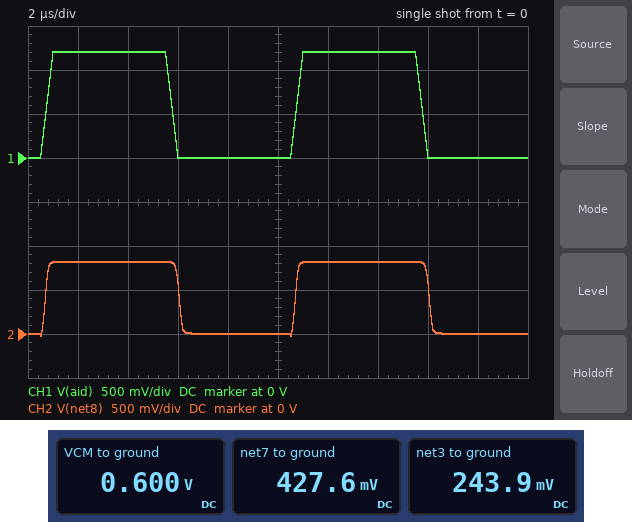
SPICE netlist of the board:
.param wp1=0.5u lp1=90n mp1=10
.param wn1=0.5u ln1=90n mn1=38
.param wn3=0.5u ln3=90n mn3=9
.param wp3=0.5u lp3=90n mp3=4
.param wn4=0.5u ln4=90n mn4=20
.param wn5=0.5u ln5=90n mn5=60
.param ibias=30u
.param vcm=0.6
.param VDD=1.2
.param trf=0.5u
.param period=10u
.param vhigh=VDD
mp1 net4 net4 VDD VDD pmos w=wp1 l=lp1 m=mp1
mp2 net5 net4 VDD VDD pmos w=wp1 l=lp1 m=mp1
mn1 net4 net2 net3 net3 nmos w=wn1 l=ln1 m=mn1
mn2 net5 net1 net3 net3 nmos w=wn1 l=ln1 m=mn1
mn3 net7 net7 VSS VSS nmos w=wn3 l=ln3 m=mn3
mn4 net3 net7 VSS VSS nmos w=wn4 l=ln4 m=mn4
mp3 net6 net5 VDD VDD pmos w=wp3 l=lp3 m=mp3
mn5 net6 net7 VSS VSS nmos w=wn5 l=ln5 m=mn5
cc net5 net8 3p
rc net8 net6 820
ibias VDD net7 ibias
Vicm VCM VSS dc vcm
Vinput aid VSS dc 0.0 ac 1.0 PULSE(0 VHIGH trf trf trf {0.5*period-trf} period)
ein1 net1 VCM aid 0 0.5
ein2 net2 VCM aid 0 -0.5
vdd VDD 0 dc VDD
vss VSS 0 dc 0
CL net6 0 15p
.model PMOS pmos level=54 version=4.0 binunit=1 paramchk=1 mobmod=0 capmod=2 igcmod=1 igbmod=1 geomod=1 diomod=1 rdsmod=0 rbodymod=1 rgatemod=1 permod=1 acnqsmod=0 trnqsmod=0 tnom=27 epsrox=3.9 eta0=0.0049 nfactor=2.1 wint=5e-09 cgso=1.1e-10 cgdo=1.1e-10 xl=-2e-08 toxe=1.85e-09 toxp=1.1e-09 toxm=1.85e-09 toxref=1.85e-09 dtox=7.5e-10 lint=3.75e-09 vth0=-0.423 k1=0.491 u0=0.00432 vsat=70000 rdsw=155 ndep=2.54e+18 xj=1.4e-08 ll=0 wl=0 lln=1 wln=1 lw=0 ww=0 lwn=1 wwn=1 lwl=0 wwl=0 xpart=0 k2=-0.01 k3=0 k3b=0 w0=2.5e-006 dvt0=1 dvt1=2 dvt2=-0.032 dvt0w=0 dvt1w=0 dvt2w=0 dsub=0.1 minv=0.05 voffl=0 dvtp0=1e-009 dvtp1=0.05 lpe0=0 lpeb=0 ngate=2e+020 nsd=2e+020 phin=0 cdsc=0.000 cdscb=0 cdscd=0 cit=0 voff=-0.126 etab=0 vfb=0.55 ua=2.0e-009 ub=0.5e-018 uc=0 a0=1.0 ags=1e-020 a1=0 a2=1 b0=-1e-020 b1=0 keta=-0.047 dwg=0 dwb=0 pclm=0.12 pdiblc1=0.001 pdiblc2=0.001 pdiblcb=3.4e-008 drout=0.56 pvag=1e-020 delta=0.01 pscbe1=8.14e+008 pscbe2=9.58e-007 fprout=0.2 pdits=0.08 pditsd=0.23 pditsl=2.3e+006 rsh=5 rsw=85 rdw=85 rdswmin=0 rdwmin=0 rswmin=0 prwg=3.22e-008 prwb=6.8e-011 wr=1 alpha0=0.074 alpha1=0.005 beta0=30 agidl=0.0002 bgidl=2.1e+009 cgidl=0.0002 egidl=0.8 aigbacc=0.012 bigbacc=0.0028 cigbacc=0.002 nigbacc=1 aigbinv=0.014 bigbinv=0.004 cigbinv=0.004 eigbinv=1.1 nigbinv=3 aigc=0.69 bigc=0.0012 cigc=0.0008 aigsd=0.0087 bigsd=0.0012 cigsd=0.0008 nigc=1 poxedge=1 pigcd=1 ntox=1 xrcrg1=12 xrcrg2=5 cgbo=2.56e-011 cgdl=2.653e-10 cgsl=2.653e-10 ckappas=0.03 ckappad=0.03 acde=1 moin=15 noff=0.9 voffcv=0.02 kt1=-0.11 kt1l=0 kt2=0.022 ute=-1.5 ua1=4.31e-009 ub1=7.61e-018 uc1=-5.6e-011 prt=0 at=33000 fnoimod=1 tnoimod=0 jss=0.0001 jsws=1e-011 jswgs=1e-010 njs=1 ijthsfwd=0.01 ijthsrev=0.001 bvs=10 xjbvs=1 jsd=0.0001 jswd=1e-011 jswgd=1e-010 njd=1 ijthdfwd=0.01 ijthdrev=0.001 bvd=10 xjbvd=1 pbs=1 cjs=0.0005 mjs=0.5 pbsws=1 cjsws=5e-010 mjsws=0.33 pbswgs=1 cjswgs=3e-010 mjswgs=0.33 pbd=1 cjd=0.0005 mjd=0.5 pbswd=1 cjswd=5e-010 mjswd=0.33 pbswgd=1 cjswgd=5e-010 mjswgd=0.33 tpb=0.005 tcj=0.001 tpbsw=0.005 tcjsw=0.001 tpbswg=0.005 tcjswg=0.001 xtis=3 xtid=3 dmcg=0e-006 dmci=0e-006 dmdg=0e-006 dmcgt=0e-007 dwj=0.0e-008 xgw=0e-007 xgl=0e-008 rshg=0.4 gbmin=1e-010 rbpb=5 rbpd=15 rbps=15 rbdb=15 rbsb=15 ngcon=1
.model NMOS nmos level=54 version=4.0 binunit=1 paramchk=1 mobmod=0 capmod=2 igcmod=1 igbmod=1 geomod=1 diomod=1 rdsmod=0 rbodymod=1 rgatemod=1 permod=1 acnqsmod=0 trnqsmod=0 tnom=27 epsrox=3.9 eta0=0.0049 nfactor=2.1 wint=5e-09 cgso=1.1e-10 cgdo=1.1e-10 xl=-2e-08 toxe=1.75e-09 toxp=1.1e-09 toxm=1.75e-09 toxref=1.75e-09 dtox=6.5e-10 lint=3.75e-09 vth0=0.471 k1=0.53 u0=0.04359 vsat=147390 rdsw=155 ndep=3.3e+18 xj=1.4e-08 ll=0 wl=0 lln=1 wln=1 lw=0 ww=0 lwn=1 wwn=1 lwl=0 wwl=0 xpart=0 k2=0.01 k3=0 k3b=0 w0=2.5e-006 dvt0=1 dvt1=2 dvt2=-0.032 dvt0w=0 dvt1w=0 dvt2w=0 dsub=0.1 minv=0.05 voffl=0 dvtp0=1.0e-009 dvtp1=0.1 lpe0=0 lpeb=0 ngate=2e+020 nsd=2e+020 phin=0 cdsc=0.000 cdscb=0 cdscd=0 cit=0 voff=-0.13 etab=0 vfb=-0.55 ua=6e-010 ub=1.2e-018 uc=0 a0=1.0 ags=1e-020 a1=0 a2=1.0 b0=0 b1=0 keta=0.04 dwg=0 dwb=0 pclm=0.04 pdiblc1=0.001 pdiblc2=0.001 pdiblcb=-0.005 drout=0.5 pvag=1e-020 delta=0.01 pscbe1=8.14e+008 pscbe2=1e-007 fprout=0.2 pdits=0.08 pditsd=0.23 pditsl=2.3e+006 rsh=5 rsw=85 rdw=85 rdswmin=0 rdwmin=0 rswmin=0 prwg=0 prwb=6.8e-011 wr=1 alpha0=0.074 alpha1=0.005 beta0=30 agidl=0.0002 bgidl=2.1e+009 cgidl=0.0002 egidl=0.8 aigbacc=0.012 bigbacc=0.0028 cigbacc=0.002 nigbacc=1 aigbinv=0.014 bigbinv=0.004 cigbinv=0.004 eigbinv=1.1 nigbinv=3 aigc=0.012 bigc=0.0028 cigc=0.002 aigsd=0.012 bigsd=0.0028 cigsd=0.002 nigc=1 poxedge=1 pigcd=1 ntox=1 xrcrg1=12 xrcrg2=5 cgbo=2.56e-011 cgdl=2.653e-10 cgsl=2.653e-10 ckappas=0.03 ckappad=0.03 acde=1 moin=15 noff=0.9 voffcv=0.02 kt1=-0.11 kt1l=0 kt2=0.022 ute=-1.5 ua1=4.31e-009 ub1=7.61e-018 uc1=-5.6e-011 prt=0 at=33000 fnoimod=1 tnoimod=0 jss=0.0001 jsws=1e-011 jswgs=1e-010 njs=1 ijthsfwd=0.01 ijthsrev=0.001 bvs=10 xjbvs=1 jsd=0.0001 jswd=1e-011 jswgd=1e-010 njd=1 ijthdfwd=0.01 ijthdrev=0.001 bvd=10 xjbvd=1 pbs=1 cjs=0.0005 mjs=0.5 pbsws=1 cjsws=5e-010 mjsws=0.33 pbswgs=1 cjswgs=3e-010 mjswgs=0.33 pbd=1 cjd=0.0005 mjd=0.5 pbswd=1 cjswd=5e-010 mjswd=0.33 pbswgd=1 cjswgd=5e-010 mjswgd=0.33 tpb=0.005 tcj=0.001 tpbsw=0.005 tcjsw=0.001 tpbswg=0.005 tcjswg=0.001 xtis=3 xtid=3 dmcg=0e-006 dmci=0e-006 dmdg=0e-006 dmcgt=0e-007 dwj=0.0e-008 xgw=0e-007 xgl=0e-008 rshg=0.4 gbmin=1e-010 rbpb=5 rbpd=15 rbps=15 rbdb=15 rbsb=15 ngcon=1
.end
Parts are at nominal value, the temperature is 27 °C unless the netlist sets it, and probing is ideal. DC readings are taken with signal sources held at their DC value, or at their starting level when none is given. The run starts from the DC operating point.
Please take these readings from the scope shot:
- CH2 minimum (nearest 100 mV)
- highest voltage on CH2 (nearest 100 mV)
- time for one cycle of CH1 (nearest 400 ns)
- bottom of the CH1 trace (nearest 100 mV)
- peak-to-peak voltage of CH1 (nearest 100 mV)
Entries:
0 V
800 mV
10.0 µs
0 V
1.2 V
